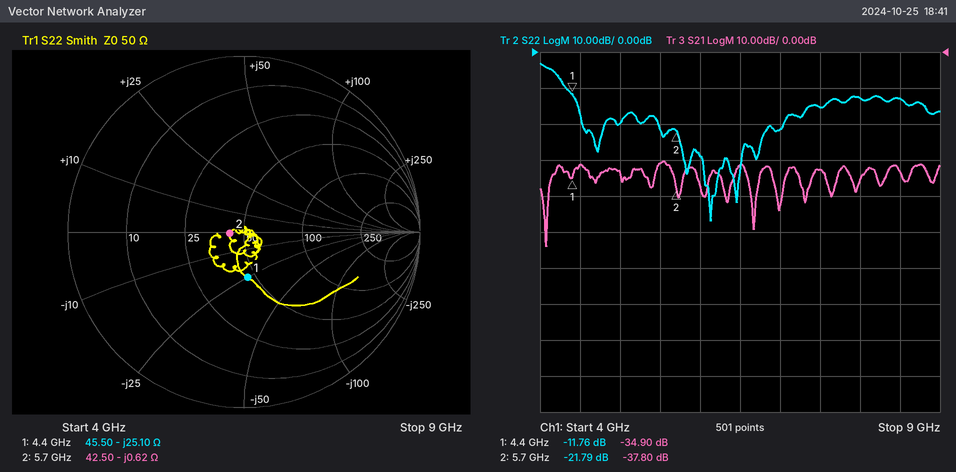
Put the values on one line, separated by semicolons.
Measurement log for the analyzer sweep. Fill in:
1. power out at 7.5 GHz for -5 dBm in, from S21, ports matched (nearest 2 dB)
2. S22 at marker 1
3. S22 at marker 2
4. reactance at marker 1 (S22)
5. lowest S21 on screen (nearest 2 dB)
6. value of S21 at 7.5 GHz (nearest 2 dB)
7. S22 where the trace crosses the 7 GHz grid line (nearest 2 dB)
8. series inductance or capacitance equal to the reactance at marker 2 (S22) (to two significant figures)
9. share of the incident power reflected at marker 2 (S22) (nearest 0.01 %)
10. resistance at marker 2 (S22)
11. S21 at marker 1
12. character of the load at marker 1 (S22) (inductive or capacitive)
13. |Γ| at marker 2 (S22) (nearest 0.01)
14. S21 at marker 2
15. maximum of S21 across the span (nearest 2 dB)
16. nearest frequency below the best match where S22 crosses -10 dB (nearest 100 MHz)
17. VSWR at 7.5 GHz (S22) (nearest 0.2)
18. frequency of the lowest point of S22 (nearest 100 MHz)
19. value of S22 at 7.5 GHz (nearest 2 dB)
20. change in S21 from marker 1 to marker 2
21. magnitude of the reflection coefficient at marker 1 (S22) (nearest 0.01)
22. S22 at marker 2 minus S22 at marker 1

-38 dBm; -11.76 dB; -21.79 dB; -25.10 Ω; -54 dB; -32 dB; -22 dB; 45 pF; 0.66 %; 42.50 Ω; -34.90 dB; capacitive; 0.08; -37.80 dB; -30 dB; 4.3 GHz; 1.4; 6.1 GHz; -16 dB; -2.90 dB; 0.26; -10.03 dB
